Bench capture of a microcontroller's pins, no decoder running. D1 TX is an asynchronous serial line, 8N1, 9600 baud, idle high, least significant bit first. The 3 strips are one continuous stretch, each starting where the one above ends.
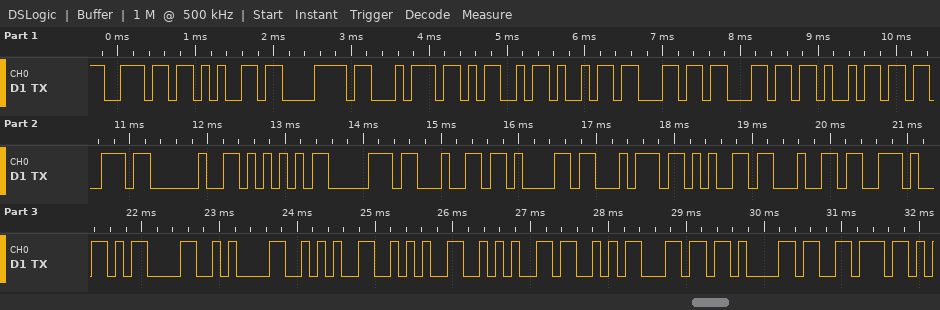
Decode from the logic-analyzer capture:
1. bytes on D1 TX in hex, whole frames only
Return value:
6E 65 78 74 4D 69 6C 6C 69 73 20 55 70 64 61 74 65 64 2E 0D 0A 2A 2A 2A 53 6C 61 76
